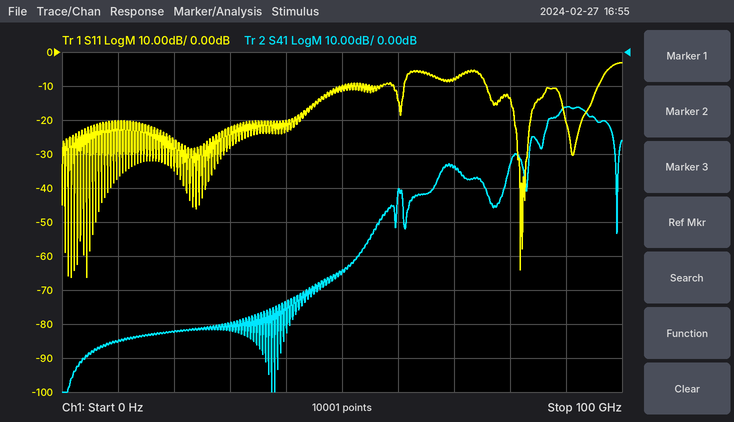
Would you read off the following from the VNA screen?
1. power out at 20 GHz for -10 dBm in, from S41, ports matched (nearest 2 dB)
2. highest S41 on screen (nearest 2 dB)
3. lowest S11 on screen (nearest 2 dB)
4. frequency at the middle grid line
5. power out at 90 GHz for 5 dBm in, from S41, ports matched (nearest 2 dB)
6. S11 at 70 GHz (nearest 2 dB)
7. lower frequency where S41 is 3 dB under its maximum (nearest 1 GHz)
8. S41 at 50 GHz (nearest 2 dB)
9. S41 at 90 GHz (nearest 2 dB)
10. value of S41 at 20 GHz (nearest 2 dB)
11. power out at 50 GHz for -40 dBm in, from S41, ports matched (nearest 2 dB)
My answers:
-92 dBm
-16 dB
-66 dB
50 GHz
-12 dBm
-8 dB
88 GHz
-64 dB
-16 dB
-82 dB
-104 dBm
